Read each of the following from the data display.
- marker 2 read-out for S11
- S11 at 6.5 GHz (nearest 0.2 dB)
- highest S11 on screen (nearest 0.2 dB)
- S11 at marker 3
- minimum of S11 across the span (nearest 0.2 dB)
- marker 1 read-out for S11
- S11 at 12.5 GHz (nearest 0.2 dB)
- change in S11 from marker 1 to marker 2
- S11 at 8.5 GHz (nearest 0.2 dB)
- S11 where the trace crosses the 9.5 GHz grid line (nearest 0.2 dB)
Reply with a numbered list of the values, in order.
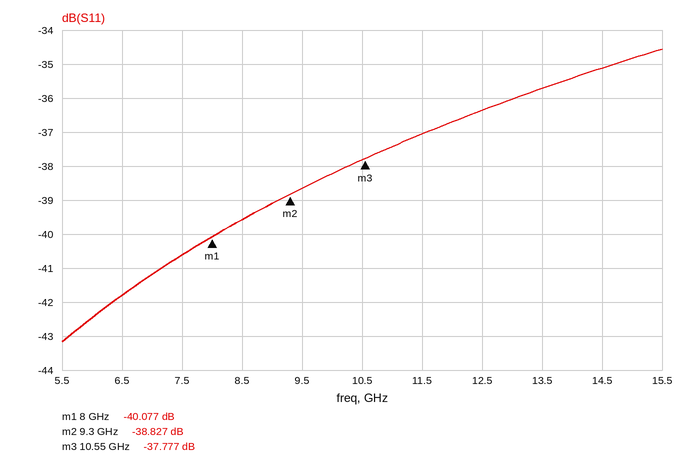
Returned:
1. -38.827 dB
2. -41.8 dB
3. -34.6 dB
4. -37.777 dB
5. -43.2 dB
6. -40.077 dB
7. -36.4 dB
8. 1.250 dB
9. -39.6 dB
10. -38.6 dB
